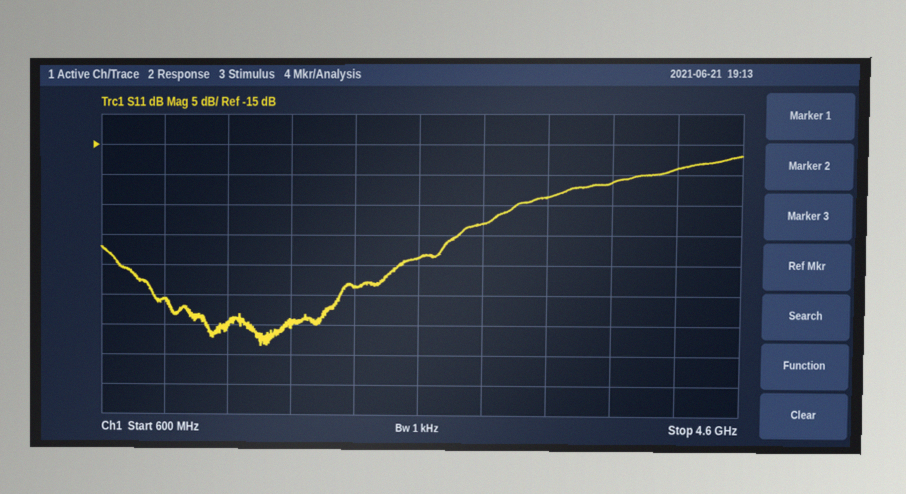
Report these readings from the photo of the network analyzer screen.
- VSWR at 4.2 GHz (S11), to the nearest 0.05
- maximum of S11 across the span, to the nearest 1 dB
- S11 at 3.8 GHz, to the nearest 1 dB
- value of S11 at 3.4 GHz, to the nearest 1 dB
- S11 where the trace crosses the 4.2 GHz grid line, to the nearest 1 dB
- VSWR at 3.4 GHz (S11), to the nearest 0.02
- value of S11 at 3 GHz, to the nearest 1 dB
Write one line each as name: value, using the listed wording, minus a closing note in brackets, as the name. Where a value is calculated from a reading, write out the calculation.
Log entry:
VSWR at 4.2 GHz (S11), to the nearest 0.05: |Γ| = 10^(-19/20) = 0.1122; VSWR = (1 + 0.1122)/(1 − 0.1122) ≈ 1.25
maximum of S11 across the span, to the nearest 1 dB: -17 dB
S11 at 3.8 GHz, to the nearest 1 dB: -21 dB
value of S11 at 3.4 GHz, to the nearest 1 dB: -24 dB
S11 where the trace crosses the 4.2 GHz grid line, to the nearest 1 dB: -19 dB
VSWR at 3.4 GHz (S11), to the nearest 0.02: |Γ| = 10^(-24/20) = 0.0631; VSWR = (1 + 0.0631)/(1 − 0.0631) ≈ 1.13, so 1.14 to the nearest 0.02
value of S11 at 3 GHz, to the nearest 1 dB: -28 dB
